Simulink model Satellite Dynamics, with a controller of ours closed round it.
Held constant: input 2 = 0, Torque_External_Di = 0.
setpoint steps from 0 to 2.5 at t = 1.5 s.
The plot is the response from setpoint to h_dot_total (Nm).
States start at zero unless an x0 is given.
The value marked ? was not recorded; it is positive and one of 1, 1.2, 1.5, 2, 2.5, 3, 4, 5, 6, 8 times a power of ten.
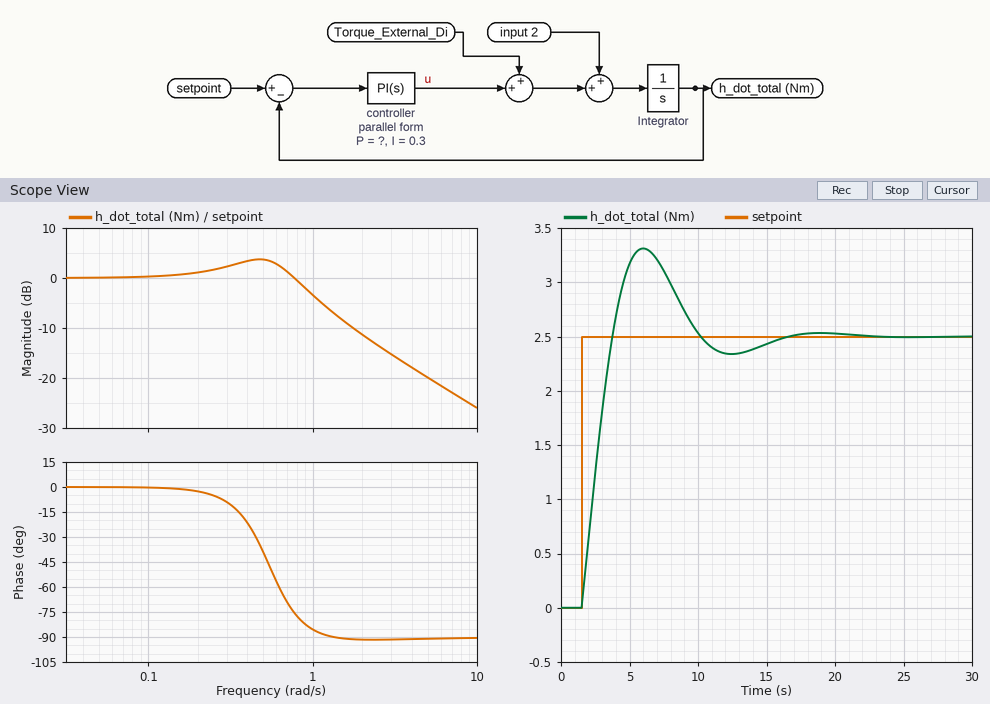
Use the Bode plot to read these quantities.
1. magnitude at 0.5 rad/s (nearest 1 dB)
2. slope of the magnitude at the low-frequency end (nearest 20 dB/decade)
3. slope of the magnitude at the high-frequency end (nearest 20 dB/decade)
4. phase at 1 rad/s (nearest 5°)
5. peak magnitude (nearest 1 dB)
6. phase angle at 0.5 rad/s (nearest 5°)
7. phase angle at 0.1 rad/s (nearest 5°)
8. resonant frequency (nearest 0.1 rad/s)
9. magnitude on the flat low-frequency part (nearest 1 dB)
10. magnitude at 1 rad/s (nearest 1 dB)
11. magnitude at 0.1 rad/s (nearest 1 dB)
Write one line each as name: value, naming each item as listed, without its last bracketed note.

magnitude at 0.5 rad/s: 4 dB
slope of the magnitude at the low-frequency end: 0 dB/decade
slope of the magnitude at the high-frequency end: -20 dB/decade
phase at 1 rad/s: -85°
peak magnitude: 4 dB
phase angle at 0.5 rad/s: -40°
phase angle at 0.1 rad/s: 0°
resonant frequency: 0.5 rad/s
magnitude on the flat low-frequency part: 0 dB
magnitude at 1 rad/s: -3 dB
magnitude at 0.1 rad/s: 0 dB
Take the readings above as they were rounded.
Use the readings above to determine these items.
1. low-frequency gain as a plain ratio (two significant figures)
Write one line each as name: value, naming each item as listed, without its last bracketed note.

low-frequency gain as a plain ratio: 1.0
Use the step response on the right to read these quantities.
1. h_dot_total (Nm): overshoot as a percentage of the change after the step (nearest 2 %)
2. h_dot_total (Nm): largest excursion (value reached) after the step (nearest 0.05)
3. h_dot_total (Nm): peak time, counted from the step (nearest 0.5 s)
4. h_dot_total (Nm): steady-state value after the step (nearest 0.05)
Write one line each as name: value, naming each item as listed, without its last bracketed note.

h_dot_total (Nm): overshoot as a percentage of the change after the step: 32 %
h_dot_total (Nm): largest excursion (value reached) after the step: 3.30
h_dot_total (Nm): peak time, counted from the step: 4.5 s
h_dot_total (Nm): steady-state value after the step: 2.50
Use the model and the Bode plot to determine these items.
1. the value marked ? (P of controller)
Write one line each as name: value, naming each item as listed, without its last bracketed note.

the value marked ?: 0.5
